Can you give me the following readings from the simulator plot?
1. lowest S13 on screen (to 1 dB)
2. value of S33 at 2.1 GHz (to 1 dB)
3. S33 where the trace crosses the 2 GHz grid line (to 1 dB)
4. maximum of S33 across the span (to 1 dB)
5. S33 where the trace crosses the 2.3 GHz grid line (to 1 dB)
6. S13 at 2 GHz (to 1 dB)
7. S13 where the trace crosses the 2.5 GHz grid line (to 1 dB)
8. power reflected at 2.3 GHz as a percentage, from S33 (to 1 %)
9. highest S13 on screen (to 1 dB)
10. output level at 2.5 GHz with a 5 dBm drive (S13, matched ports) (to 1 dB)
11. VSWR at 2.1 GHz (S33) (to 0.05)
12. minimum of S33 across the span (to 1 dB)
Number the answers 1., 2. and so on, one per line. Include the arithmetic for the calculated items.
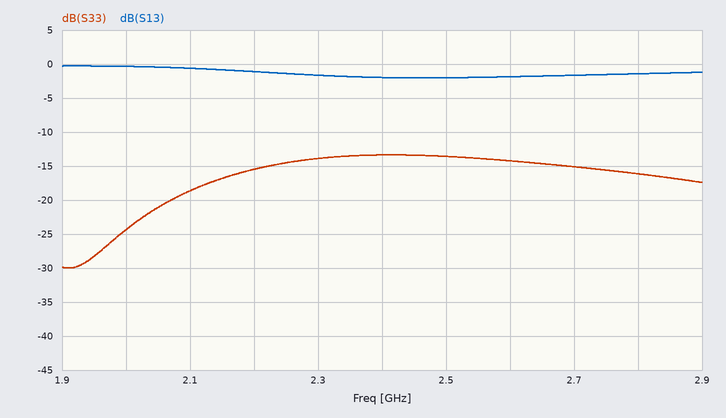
1. -2 dB
2. -19 dB
3. -24 dB
4. -13 dB
5. -14 dB
6. 0 dB
7. -2 dB
8. 10^(-14/10) ≈ 4 %
9. 0 dB
10. 5 dBm + (-2 dB) = 3 dBm
11. |Γ| = 10^(-19/20) = 0.1122; VSWR = (1 + 0.1122)/(1 − 0.1122) ≈ 1.25
12. -30 dB
